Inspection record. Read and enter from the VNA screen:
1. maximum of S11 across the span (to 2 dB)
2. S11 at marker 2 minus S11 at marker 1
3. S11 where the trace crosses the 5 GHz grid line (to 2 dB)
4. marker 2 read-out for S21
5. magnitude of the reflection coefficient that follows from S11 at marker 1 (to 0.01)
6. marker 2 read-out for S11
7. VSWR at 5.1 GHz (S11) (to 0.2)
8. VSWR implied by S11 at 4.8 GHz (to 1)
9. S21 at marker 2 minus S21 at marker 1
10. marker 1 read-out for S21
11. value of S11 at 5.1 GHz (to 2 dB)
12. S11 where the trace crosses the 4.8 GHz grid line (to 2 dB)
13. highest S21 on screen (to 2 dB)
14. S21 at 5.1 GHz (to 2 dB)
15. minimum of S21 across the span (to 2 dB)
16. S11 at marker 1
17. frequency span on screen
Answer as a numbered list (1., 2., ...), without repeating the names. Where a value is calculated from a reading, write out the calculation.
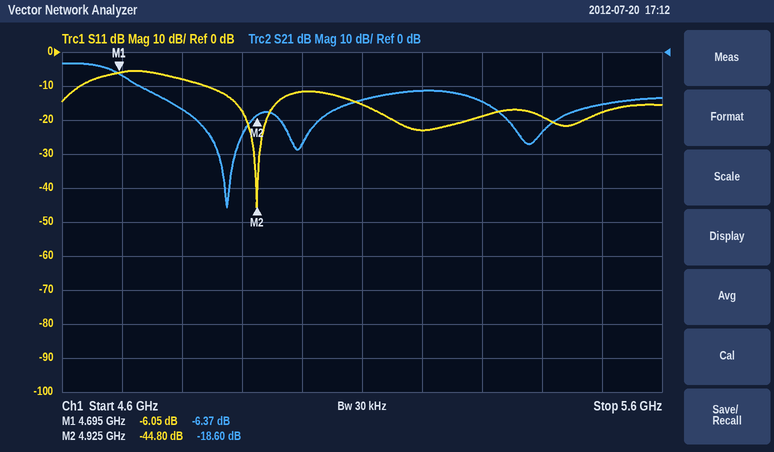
1. -6 dB
2. -44.8 − (-6.05) = -38.75 dB
3. -12 dB
4. -18.60 dB
5. 10^(-6.05/20) ≈ 0.50
6. -44.80 dB
7. |Γ| = 10^(-16/20) = 0.1585; VSWR = (1 + 0.1585)/(1 − 0.1585) ≈ 1.4
8. |Γ| = 10^(-8/20) = 0.3981; VSWR = (1 + 0.3981)/(1 − 0.3981) ≈ 2
9. -18.6 − (-6.37) = -12.23 dB
10. -6.37 dB
11. -16 dB
12. -8 dB
13. -4 dB
14. -14 dB
15. -46 dB
16. -6.05 dB
17. 1 GHz
